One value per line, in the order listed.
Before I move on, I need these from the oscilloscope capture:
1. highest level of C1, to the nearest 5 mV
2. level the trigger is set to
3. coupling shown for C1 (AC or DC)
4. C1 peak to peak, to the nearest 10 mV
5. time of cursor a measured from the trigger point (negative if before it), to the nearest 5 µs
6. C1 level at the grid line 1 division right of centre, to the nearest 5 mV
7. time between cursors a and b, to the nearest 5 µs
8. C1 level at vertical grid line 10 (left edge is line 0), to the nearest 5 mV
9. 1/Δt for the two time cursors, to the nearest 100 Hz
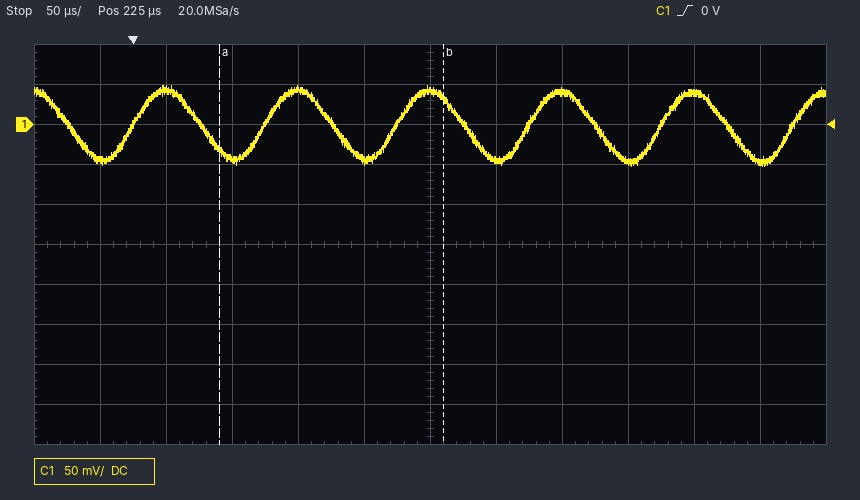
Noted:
50 mV
0 V
DC
100 mV
+65 µs
-45 mV
170 µs
40 mV
5.9 kHz
